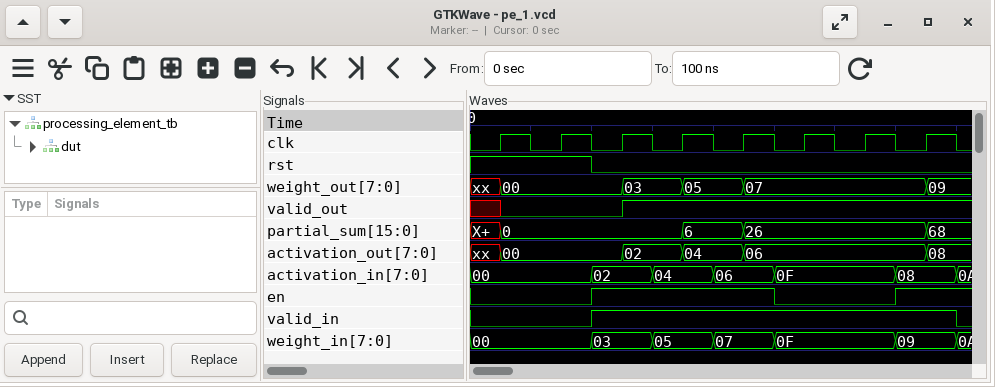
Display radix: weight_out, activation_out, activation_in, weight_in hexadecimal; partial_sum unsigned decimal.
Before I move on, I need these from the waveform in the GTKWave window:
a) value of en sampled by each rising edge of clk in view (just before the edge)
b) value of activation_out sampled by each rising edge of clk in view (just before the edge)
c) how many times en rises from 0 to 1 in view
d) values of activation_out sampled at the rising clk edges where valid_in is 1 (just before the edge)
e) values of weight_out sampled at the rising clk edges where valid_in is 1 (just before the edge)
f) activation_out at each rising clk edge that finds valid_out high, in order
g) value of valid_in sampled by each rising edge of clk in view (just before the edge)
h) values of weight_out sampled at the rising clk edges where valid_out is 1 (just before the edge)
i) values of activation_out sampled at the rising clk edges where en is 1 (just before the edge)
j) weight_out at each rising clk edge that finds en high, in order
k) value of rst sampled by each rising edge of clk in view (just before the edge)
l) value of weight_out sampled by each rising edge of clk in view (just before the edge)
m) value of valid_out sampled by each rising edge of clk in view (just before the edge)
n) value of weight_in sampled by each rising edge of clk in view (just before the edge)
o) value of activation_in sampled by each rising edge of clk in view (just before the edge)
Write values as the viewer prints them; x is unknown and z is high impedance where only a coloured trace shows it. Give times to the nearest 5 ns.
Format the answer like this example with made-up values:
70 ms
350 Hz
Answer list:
0 0 1 1 1 0 0 1
xx, 00, 00, 02, 04, 06, 06, 06
2
00, 02, 04, 06, 06, 06
00, 03, 05, 07, 07, 07
02, 04, 06, 06, 06
0 0 1 1 1 1 1 1
03, 05, 07, 07, 07
00, 02, 04, 06
00, 03, 05, 07
1 1 0 0 0 0 0 0
xx, 00, 00, 03, 05, 07, 07, 07
x 0 0 1 1 1 1 1
00, 00, 03, 05, 07, 0F, 0F, 09
00, 00, 02, 04, 06, 0F, 0F, 08
